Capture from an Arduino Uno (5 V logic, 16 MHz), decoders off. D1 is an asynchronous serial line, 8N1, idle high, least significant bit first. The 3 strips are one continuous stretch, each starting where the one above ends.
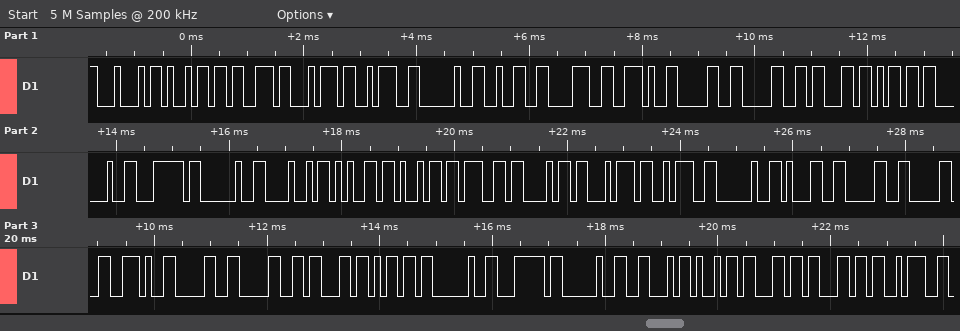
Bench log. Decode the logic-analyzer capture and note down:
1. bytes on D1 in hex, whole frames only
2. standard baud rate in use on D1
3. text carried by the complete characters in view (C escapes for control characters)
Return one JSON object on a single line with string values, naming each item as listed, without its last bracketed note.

{"bytes on D1 in hex, whole frames only": "44 69 73 74 3A 20 32 38 2E 30 30 63 6D 20 7C 20 48 65 69 67 68 74 3A 20 31 30 30 2E 30 30 63 6D 20 7C 20 46 69 6C 6C 3A", "standard baud rate in use on D1": "9600 baud", "text carried by the complete characters in view": "\"Dist: 28.00cm | Height: 100.00cm | Fill:\""}
